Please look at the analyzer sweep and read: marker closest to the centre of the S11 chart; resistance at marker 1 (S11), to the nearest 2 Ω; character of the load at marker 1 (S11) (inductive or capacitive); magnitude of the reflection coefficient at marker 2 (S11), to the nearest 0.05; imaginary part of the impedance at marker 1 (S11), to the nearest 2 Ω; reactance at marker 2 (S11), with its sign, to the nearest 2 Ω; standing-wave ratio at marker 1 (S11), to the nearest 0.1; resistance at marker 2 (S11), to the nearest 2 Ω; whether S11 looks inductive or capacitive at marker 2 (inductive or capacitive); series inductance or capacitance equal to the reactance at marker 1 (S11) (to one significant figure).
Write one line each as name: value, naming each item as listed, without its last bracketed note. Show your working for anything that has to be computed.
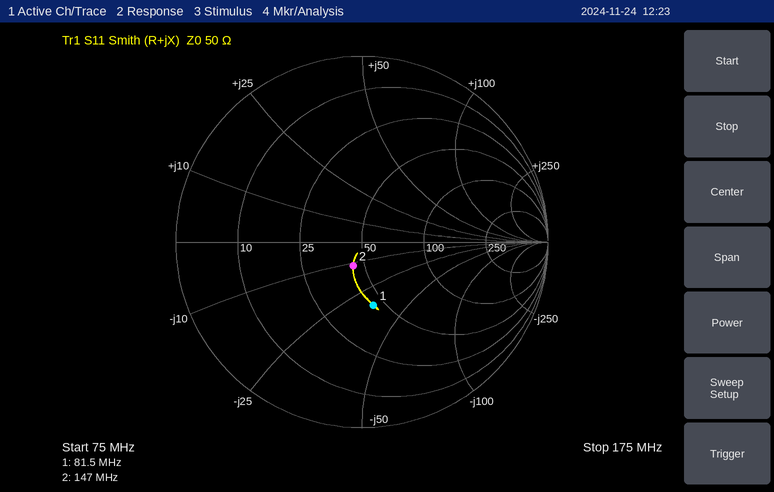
marker closest to the centre of the S11 chart: marker 2
resistance at marker 1 (S11), to the nearest 2 Ω: 44 Ω
character of the load at marker 1 (S11): capacitive
magnitude of the reflection coefficient at marker 2 (S11), to the nearest 0.05: 0.15
imaginary part of the impedance at marker 1 (S11), to the nearest 2 Ω: -34 Ω
reactance at marker 2 (S11), with its sign, to the nearest 2 Ω: -12 Ω
standing-wave ratio at marker 1 (S11), to the nearest 0.1: 2.1
resistance at marker 2 (S11), to the nearest 2 Ω: 44 Ω
whether S11 looks inductive or capacitive at marker 2: capacitive
series inductance or capacitance equal to the reactance at marker 1 (S11): C = 1/(2π × 81.5 MHz × 34 Ω) ≈ 57.4 pF, so 60 pF to one significant figure
